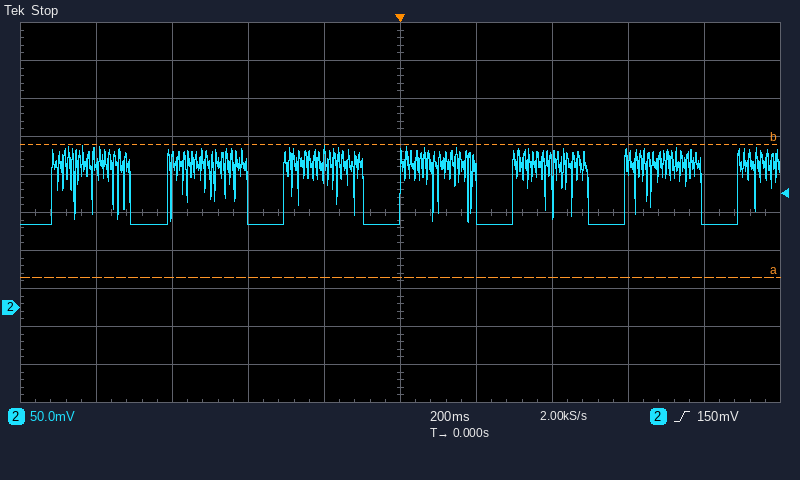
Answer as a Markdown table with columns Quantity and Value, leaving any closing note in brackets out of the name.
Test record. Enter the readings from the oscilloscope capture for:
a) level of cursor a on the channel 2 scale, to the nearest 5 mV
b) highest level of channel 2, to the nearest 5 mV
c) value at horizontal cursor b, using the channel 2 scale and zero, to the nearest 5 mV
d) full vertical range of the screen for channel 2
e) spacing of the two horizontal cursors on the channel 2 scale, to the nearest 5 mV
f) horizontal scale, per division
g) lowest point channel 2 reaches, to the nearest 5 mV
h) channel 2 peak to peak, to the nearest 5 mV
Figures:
| Quantity | Value |
|---|---|
| level of cursor a on the channel 2 scale, to the nearest 5 mV | 40 mV |
| highest level of channel 2, to the nearest 5 mV | 215 mV |
| value at horizontal cursor b, using the channel 2 scale and zero, to the nearest 5 mV | 215 mV |
| full vertical range of the screen for channel 2 | 500 mV |
| spacing of the two horizontal cursors on the channel 2 scale, to the nearest 5 mV | 175 mV |
| horizontal scale, per division | 200 ms |
| lowest point channel 2 reaches, to the nearest 5 mV | 110 mV |
| channel 2 peak to peak, to the nearest 5 mV | 105 mV |
